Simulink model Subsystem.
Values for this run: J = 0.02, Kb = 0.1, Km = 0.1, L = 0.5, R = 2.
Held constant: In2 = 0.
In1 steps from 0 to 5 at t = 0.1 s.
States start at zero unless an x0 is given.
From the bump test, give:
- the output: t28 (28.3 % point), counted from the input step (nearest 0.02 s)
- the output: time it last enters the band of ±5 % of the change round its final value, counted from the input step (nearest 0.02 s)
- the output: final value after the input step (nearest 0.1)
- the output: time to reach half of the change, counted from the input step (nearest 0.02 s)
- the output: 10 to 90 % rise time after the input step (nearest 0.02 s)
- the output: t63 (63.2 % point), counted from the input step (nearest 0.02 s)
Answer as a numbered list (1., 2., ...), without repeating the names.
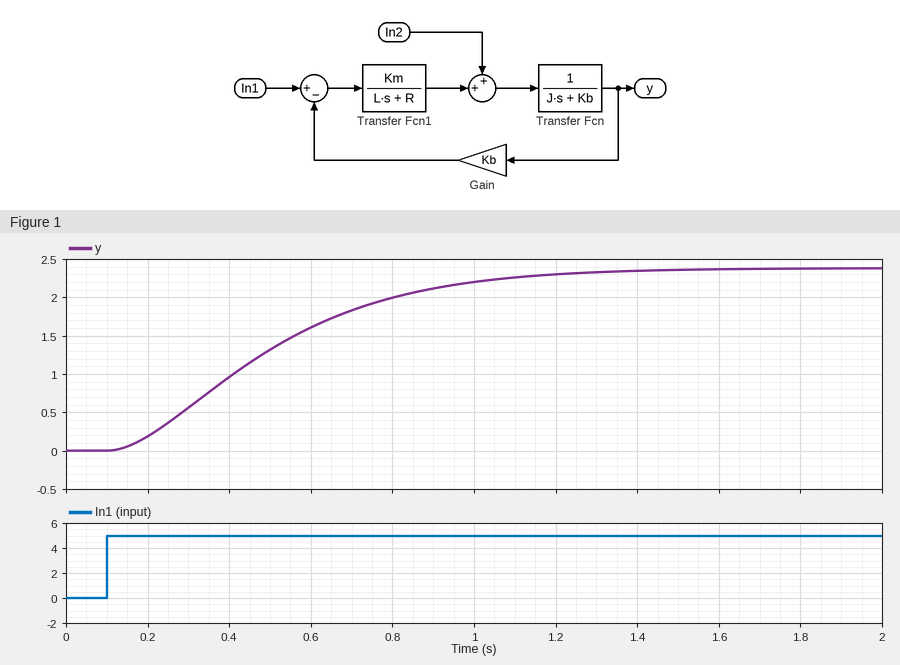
1. 0.22 s
2. 1.00 s
3. 2.4
4. 0.36 s
5. 0.72 s
6. 0.46 s
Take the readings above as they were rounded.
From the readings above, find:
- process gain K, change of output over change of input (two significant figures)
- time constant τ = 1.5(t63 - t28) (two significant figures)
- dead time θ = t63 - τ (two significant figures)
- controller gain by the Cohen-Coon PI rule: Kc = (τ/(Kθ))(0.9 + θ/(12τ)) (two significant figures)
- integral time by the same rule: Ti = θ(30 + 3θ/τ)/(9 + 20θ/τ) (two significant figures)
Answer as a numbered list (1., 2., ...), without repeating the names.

1. 0.48
2. 0.36 s
3. 0.10 s
4. 6.9
5. 0.21 s
